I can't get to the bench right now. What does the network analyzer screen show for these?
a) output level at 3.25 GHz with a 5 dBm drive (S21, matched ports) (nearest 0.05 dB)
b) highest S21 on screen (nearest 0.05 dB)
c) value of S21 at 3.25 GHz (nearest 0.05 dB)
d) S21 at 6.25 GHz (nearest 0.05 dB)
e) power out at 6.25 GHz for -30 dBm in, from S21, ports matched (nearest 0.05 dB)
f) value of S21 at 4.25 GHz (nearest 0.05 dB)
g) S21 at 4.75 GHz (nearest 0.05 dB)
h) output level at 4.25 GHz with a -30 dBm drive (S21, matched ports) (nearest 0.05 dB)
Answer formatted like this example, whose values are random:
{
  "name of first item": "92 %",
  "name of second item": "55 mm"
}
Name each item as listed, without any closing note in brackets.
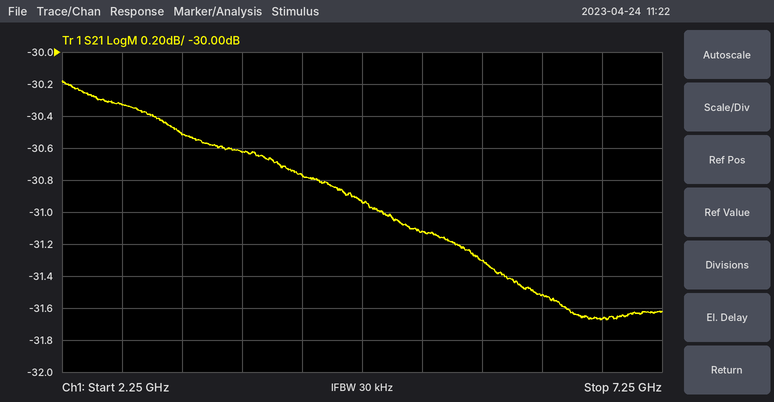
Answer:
{
  "output level at 3.25 GHz with a 5 dBm drive (S21, matched ports)": "-25.50 dBm",
  "highest S21 on screen": "-30.20 dB",
  "value of S21 at 3.25 GHz": "-30.50 dB",
  "S21 at 6.25 GHz": "-31.50 dB",
  "power out at 6.25 GHz for -30 dBm in, from S21, ports matched": "-61.50 dBm",
  "value of S21 at 4.25 GHz": "-30.75 dB",
  "S21 at 4.75 GHz": "-30.95 dB",
  "output level at 4.25 GHz with a -30 dBm drive (S21, matched ports)": "-60.75 dBm"
}
